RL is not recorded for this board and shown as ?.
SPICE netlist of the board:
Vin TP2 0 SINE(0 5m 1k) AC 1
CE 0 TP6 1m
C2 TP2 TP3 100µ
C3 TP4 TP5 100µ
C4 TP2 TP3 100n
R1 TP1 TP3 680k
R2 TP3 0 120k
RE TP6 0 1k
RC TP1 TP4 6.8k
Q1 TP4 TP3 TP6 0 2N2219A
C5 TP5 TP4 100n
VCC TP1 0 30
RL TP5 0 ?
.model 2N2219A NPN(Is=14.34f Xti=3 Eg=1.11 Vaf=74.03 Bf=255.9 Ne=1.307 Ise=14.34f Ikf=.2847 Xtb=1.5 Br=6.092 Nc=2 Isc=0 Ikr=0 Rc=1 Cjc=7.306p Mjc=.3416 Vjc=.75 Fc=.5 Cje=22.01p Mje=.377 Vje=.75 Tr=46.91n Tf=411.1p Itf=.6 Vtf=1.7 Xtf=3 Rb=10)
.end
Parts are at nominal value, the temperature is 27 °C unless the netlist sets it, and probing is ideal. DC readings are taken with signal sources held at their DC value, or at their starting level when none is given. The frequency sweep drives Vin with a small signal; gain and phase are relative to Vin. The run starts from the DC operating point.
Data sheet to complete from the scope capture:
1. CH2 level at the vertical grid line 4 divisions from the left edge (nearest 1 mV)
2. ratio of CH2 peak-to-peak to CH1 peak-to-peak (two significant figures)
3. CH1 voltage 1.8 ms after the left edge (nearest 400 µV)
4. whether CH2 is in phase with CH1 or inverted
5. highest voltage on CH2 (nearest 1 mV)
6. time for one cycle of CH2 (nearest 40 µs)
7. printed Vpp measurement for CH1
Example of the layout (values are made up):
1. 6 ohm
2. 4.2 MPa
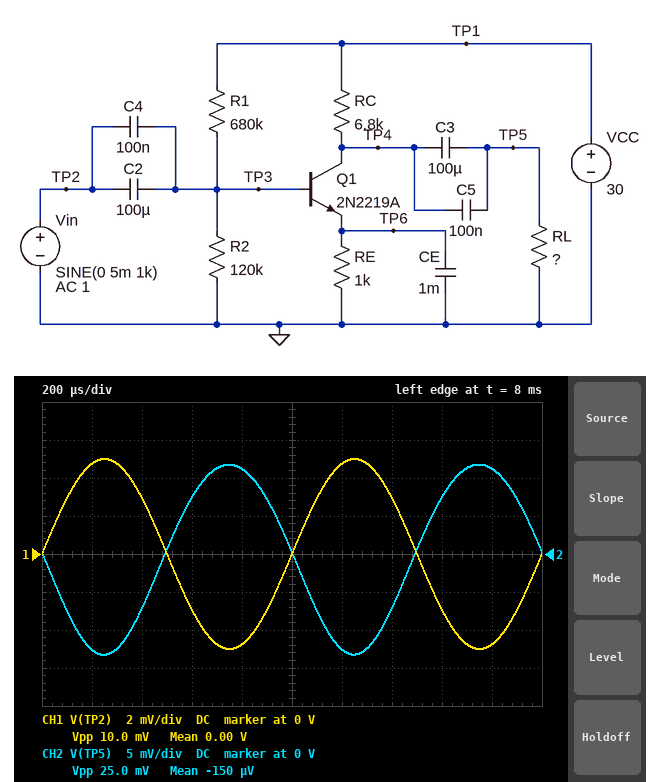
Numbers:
1. 11 mV
2. 2.5
3. -4.8 mV
4. inverted
5. 12 mV
6. 1.00 ms
7. 10.0 mV
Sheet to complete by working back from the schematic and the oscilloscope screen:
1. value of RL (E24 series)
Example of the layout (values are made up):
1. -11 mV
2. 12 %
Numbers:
1. 27 Ω
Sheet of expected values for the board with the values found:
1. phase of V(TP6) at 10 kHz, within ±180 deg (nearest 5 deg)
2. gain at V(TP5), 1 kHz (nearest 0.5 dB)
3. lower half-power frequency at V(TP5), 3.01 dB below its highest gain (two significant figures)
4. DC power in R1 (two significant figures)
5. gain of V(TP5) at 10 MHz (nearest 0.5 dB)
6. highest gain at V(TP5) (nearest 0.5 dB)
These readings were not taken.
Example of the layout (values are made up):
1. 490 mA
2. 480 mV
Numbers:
1. -90 deg
2. 8.0 dB
3. 16 Hz
4. 1.1 mW
5. 8.0 dB
6. 8.0 dB
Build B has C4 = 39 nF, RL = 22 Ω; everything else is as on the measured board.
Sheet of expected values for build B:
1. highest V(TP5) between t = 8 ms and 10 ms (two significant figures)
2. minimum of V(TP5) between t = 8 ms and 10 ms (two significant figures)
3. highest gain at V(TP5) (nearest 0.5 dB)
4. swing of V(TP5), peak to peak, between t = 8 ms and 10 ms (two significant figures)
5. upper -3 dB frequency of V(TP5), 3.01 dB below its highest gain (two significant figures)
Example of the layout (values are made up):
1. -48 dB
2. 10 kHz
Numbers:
1. 9.6 mV
2. -11 mV
3. 6.0 dB
4. 20 mV
5. 190 MHz
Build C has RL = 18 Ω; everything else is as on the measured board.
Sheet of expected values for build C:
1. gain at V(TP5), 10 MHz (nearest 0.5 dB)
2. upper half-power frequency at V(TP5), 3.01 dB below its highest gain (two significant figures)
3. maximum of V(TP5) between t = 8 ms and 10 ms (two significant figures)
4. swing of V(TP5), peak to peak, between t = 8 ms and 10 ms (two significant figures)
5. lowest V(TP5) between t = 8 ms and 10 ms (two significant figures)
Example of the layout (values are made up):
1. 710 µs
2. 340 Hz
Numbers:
1. 4.5 dB
2. 190 MHz
3. 7.9 mV
4. 17 mV
5. -8.9 mV
